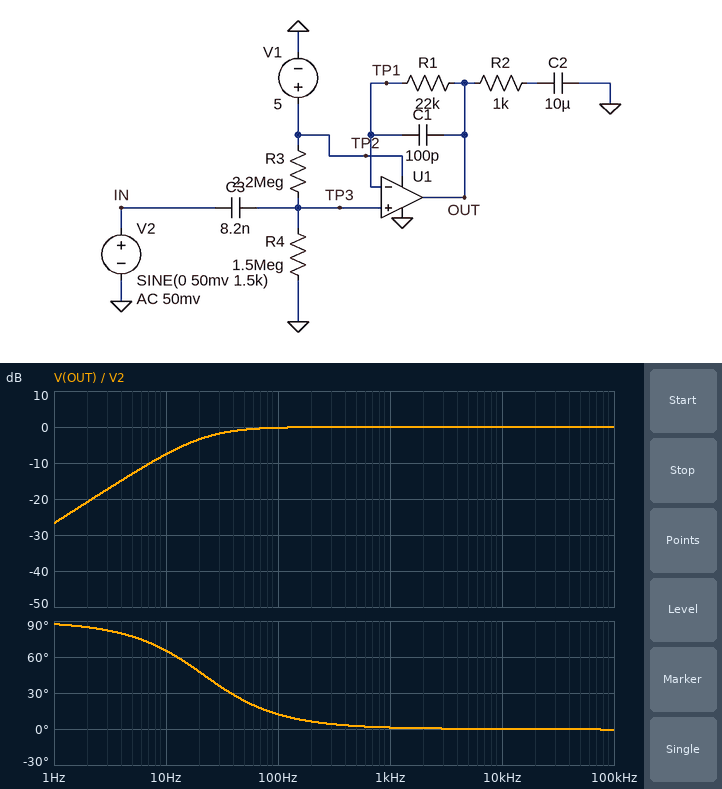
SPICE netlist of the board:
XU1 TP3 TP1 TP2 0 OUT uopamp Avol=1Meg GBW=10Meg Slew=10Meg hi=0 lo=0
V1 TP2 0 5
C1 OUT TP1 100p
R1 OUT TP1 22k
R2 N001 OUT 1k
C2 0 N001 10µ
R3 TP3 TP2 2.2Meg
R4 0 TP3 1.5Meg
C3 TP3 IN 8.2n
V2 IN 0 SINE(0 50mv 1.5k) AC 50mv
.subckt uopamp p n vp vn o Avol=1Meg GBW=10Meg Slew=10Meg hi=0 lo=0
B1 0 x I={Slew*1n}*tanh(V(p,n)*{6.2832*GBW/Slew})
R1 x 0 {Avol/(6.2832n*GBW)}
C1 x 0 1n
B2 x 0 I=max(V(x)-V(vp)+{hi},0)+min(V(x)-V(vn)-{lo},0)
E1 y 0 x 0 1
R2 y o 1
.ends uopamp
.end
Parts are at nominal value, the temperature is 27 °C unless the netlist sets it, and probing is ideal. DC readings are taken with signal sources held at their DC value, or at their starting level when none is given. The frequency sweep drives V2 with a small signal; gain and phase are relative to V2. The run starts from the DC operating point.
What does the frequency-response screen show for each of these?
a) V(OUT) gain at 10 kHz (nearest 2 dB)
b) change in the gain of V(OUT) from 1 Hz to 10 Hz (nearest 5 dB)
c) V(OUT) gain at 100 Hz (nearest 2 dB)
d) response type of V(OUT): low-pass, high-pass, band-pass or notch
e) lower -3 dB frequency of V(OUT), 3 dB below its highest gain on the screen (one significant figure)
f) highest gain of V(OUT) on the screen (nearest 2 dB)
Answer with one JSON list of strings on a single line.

["0 dB", "20 dB", "0 dB", "high-pass", "20 Hz", "0 dB"]
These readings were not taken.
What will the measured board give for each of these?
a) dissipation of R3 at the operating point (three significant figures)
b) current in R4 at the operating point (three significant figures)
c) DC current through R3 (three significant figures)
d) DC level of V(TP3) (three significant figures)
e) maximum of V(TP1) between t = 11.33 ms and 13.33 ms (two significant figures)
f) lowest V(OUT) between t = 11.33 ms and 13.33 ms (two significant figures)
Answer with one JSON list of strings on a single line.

["4.02 µW", "1.35 µA", "1.35 µA", "2.03 V", "2.1 V", "2.0 V"]
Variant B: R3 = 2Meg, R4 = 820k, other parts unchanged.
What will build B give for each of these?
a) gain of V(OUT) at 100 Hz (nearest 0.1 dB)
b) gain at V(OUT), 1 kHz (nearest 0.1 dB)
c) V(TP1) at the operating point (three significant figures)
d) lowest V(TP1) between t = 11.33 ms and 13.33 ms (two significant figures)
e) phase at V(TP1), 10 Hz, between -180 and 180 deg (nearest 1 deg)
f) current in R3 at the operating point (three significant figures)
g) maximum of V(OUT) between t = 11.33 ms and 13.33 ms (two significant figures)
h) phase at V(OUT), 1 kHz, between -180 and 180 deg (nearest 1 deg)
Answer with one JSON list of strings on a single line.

["-0.5 dB", "0 dB", "1.45 V", "1.4 V", "73 deg", "1.77 µA", "1.5 V", "2 deg"]
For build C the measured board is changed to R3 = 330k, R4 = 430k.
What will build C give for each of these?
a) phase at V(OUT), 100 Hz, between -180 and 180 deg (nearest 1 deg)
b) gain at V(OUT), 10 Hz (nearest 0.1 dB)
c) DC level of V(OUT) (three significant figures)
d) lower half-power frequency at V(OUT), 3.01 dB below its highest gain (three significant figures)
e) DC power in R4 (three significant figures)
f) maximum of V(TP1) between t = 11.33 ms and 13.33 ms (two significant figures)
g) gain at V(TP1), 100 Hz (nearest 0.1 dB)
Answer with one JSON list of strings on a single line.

["46 deg", "-20.4 dB", "2.83 V", "104 Hz", "18.6 µW", "2.9 V", "-3.2 dB"]
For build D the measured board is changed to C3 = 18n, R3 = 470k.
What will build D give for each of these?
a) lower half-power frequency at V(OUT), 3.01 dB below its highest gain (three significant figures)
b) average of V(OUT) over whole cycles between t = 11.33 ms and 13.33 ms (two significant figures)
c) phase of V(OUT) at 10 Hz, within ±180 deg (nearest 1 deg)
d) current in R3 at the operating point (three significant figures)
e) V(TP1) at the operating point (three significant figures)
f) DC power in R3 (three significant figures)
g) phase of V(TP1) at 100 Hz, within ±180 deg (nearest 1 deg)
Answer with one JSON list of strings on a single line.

["24.7 Hz", "3.8 V", "68 deg", "2.54 µA", "3.81 V", "3.03 µW", "14 deg"]
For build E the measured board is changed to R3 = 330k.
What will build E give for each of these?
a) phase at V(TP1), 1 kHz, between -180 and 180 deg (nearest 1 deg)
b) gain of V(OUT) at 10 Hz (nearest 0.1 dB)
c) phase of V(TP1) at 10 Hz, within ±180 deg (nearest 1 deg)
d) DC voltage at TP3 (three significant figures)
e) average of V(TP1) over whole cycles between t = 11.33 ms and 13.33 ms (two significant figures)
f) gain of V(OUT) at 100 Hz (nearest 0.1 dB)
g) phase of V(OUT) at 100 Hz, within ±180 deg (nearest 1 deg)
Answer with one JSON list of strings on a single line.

["4 deg", "-17.2 dB", "82 deg", "4.10 V", "4.1 V", "-1.8 dB", "36 deg"]
